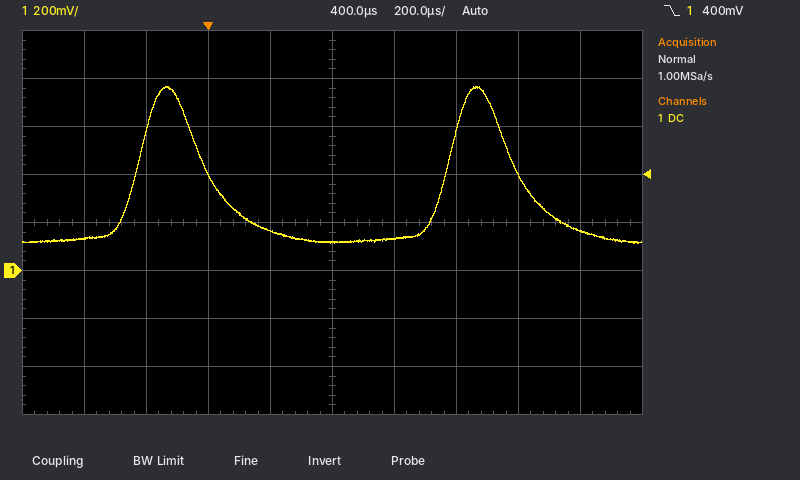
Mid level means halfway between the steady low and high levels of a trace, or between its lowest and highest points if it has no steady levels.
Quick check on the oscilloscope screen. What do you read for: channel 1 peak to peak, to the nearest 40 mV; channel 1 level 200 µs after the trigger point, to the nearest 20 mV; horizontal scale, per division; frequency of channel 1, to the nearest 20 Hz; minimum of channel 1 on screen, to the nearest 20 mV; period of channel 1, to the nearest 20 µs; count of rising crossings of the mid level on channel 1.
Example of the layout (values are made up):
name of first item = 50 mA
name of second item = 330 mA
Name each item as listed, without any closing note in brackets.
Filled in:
channel 1 peak to peak, to the nearest 40 mV = 640 mV
channel 1 level 200 µs after the trigger point, to the nearest 20 mV = 160 mV
horizontal scale, per division = 200 µs
frequency of channel 1, to the nearest 20 Hz = 1.00 kHz
minimum of channel 1 on screen, to the nearest 20 mV = 120 mV
period of channel 1, to the nearest 20 µs = 1.00 ms
count of rising crossings of the mid level on channel 1 = 2
